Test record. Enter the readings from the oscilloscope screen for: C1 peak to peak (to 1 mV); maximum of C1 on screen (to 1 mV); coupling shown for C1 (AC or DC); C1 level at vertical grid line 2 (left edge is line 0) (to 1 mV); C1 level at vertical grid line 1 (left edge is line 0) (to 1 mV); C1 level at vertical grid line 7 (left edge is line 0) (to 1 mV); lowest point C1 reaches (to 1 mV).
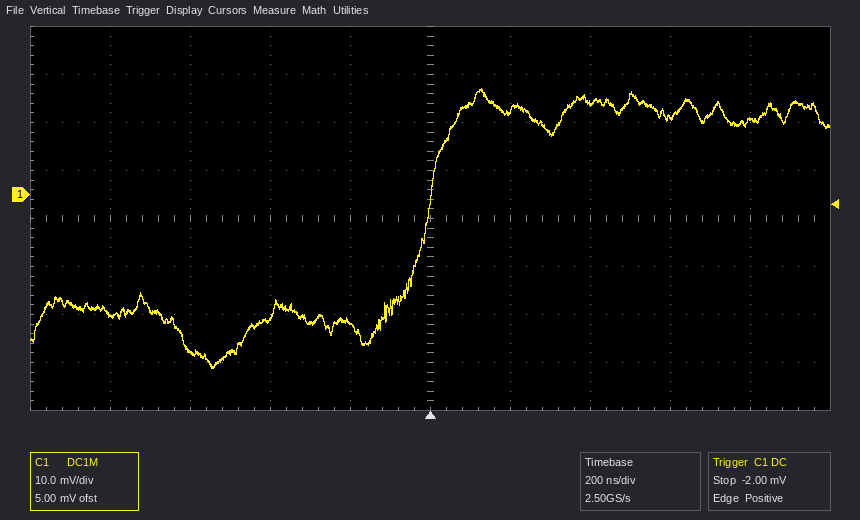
58 mV
22 mV
DC
-33 mV
-25 mV
19 mV
-36 mV
